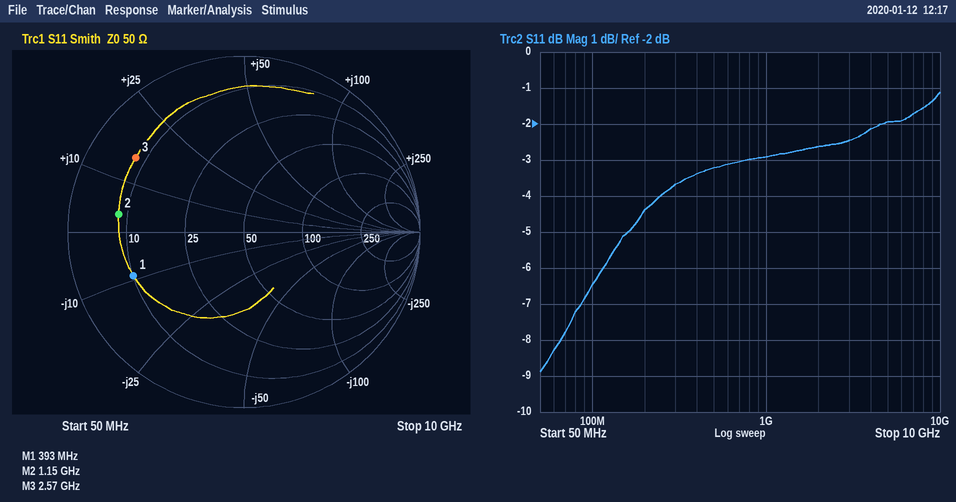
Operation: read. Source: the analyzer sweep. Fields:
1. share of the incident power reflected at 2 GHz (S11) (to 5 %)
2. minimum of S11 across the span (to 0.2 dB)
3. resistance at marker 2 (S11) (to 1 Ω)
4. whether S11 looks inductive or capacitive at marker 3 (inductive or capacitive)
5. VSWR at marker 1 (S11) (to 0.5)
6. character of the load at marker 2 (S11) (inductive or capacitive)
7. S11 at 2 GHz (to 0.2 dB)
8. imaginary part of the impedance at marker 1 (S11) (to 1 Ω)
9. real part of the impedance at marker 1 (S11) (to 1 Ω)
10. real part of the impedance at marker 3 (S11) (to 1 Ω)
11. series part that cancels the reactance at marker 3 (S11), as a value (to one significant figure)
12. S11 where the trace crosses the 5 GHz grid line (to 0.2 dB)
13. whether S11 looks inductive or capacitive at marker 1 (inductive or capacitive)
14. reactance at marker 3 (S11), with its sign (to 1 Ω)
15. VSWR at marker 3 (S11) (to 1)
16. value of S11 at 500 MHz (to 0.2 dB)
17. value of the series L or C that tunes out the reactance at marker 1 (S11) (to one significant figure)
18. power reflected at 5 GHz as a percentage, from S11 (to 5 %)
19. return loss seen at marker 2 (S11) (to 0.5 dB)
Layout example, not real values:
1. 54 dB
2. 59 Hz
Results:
1. 55 %
2. -8.8 dB
3. 8 Ω
4. inductive
5. 5.0
6. inductive
7. -2.6 dB
8. -9 Ω
9. 10 Ω
10. 8 Ω
11. 4 pF
12. -2.0 dB
13. capacitive
14. +15 Ω
15. 7
16. -3.2 dB
17. 4 nH
18. 65 %
19. 3.0 dB
